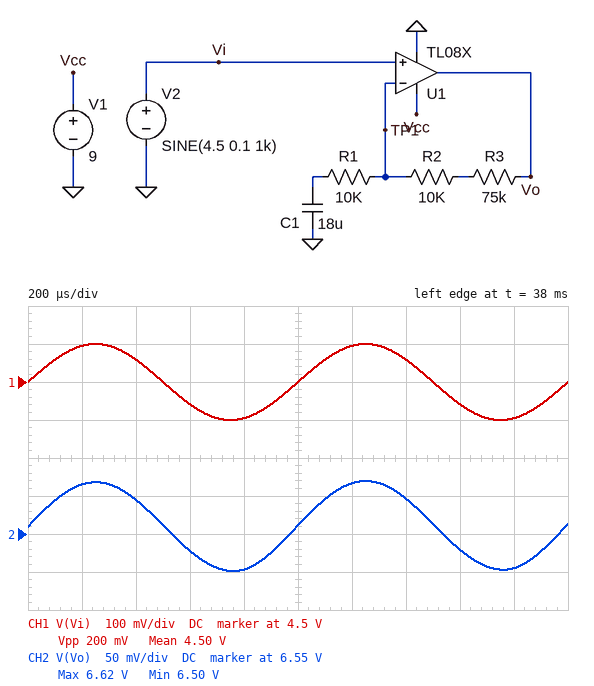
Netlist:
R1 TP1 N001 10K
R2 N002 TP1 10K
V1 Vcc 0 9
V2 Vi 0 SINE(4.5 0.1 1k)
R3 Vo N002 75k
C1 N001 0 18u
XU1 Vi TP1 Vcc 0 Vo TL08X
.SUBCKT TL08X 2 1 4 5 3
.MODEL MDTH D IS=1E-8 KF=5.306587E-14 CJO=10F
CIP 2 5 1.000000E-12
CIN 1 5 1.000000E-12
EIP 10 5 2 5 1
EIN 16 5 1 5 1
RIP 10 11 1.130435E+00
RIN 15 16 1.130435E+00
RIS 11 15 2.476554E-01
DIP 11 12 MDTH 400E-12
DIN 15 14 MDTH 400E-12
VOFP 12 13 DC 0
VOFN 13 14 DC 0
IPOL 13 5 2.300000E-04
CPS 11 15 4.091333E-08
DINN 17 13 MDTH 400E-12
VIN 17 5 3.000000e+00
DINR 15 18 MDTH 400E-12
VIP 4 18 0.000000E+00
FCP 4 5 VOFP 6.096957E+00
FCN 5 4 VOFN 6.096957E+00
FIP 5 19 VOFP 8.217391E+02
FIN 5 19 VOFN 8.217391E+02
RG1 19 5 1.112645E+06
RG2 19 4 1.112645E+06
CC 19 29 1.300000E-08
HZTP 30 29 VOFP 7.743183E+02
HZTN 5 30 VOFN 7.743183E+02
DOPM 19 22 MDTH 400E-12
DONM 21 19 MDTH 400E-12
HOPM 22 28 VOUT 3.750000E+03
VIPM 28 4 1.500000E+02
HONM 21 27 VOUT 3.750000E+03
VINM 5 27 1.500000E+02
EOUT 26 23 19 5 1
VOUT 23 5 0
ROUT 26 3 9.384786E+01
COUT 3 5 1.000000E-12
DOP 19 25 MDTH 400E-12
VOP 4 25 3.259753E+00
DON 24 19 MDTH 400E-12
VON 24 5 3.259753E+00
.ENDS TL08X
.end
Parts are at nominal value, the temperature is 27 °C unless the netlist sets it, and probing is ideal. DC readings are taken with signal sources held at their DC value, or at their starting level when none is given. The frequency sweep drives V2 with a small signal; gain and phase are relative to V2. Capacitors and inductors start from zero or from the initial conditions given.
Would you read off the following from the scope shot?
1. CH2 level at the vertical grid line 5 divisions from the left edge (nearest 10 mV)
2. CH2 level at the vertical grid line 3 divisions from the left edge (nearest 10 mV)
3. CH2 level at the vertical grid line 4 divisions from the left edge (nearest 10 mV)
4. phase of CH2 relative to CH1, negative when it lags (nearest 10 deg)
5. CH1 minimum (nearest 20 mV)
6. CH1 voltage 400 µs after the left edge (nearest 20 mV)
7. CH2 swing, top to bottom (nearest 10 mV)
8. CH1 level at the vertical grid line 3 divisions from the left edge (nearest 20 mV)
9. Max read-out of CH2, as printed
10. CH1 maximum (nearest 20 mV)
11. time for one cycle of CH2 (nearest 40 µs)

6.56 V
6.53 V
6.50 V
0 deg
4.40 V
4.56 V
120 mV
4.44 V
6.62 V
4.60 V
1.00 ms
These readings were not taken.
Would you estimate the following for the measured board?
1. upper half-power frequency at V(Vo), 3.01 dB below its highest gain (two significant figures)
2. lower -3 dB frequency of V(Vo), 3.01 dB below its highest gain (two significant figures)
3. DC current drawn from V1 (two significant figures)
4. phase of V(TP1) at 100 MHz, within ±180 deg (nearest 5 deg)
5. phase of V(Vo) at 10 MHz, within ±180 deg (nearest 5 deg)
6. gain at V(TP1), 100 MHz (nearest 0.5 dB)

510 kHz
870 mHz
1.4 mA
25 deg
-160 deg
-59.5 dB
